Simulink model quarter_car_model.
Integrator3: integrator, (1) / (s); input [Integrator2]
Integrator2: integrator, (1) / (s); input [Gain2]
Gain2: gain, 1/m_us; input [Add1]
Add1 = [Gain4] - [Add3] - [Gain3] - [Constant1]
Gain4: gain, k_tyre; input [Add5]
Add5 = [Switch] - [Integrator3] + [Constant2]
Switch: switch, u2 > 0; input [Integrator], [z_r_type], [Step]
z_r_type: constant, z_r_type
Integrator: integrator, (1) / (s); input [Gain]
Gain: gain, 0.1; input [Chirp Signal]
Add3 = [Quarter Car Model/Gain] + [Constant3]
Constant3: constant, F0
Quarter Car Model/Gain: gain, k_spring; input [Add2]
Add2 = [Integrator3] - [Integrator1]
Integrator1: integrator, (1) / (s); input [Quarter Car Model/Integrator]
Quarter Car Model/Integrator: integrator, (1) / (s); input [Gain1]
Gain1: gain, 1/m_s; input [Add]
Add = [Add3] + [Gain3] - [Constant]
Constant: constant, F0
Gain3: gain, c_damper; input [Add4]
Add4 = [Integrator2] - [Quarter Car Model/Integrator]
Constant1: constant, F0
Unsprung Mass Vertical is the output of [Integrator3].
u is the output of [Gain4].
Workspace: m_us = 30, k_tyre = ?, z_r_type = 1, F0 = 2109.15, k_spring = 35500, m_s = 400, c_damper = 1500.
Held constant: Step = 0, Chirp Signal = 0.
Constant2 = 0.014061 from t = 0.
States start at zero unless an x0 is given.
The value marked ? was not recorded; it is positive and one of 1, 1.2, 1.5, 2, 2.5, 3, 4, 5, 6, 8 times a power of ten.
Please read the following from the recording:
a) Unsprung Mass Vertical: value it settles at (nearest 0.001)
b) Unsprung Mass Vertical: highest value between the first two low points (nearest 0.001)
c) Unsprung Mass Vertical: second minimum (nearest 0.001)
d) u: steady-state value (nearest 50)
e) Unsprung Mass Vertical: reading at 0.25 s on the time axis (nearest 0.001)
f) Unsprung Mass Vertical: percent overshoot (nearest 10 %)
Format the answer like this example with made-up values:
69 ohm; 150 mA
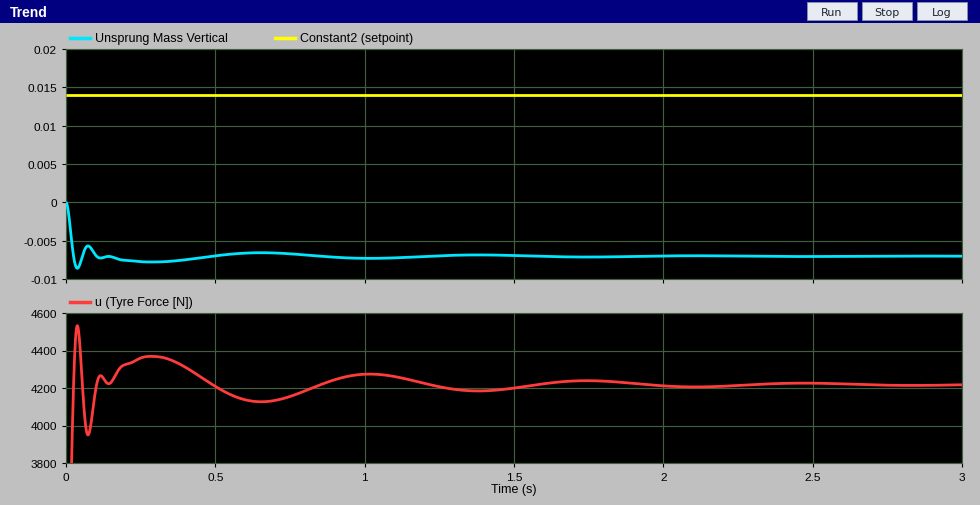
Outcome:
-0.007; -0.006; -0.008; 4200; -0.008; 20 %
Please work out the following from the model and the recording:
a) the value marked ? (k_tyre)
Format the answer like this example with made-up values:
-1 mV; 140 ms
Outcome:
200000
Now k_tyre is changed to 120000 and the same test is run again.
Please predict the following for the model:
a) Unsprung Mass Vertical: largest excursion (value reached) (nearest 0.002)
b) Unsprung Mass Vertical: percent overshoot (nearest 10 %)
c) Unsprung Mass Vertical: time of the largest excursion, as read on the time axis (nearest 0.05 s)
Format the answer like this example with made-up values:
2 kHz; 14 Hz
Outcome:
-0.024; 20 %; 0.30 s
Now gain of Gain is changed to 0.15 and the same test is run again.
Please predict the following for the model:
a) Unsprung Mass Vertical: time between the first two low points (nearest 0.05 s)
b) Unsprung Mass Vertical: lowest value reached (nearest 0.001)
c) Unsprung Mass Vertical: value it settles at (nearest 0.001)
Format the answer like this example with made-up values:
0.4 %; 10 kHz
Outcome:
0.25 s; -0.009; -0.007
